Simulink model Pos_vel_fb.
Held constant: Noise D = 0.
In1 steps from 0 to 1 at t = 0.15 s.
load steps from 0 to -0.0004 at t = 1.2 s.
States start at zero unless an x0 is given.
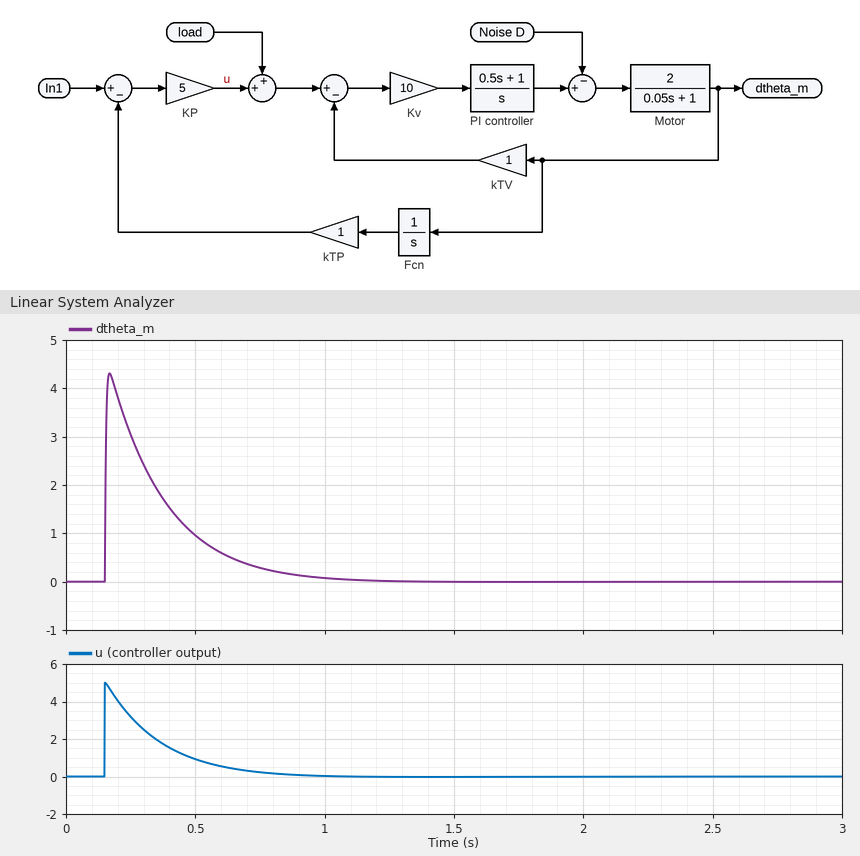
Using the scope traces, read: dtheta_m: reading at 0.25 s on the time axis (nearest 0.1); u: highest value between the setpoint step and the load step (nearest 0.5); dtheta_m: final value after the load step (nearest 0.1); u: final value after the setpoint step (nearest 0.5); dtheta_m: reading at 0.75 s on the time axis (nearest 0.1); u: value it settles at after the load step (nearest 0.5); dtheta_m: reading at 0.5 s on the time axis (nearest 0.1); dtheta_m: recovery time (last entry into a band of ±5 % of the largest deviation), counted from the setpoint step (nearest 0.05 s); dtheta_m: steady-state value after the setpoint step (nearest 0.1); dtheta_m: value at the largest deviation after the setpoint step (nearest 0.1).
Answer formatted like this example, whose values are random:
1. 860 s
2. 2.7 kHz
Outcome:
1. 3.0
2. 5.0
3. 0.0
4. 0.0
5. 0.3
6. 0.0
7. 1.0
8. 0.65 s
9. 0.0
10. 4.3
